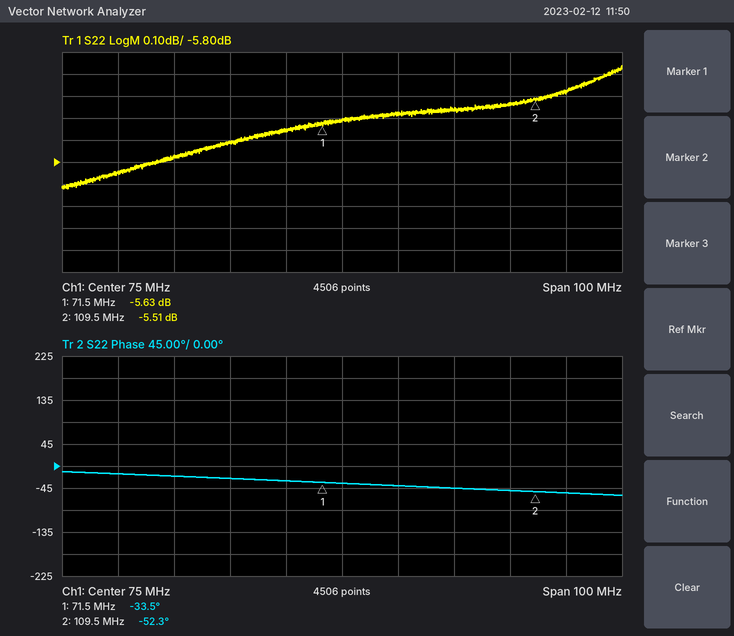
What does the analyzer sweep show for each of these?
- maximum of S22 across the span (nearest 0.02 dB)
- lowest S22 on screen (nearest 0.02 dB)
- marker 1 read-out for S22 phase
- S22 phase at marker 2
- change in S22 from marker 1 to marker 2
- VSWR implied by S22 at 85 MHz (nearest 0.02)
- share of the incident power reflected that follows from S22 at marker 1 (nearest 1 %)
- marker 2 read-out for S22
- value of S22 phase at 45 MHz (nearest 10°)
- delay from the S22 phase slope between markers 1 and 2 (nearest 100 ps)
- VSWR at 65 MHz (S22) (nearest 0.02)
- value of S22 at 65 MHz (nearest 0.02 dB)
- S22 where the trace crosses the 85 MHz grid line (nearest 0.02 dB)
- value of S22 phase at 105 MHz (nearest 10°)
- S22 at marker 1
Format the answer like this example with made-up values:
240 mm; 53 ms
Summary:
-5.36 dB; -5.92 dB; -33.5°; -52.3°; 0.12 dB; 3.22; 27 %; -5.51 dB; -20°; 1.4 ns; 3.18; -5.66 dB; -5.58 dB; -50°; -5.63 dB
